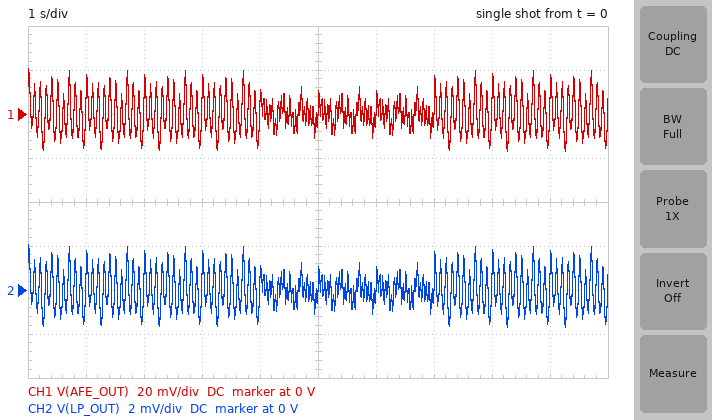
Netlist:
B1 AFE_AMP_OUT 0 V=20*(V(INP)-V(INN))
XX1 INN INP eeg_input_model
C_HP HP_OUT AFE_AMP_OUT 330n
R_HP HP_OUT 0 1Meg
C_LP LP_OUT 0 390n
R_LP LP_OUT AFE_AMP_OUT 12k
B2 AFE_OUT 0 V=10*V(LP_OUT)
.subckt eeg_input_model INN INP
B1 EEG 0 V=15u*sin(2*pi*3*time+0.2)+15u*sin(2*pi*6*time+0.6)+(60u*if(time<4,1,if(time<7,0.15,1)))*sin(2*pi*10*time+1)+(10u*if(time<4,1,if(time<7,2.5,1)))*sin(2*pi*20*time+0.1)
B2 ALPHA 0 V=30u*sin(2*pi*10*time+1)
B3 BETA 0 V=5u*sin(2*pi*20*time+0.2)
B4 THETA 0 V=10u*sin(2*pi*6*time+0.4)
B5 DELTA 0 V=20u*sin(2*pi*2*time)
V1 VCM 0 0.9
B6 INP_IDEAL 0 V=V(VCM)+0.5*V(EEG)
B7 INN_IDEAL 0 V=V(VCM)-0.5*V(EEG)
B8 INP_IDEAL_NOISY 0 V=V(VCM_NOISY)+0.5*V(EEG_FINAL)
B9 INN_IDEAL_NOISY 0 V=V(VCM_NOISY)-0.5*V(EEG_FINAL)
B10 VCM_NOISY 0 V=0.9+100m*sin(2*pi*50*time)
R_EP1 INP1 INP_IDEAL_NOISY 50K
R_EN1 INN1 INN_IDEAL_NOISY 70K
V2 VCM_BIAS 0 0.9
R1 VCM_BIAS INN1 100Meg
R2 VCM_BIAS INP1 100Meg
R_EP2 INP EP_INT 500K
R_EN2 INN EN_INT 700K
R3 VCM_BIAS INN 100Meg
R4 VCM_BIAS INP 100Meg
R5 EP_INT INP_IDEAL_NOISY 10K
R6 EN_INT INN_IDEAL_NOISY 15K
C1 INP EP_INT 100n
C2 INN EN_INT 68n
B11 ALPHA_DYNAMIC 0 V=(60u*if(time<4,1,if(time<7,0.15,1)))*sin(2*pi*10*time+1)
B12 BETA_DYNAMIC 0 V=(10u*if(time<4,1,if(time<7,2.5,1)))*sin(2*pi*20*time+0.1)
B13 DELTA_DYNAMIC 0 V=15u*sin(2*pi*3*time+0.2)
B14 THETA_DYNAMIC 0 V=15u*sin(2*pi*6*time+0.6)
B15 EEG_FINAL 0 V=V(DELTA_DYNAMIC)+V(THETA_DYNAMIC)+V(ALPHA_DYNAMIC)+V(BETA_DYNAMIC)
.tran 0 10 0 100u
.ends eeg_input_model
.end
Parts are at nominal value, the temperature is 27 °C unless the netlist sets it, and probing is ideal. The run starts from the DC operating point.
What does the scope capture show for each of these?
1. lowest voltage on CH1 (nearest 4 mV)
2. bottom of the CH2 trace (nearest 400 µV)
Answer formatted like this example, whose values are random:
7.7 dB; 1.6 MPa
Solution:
-16 mV; -1.6 mV
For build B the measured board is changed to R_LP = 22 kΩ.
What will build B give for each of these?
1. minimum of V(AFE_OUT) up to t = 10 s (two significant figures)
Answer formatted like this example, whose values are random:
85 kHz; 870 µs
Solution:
-15 mV
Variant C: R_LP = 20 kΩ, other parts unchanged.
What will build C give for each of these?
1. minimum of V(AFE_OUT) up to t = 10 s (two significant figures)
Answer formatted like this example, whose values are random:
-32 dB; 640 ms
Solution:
-15 mV
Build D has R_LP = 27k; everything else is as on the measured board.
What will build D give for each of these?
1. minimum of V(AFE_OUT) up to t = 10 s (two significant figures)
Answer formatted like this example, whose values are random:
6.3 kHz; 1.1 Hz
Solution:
-14 mV
